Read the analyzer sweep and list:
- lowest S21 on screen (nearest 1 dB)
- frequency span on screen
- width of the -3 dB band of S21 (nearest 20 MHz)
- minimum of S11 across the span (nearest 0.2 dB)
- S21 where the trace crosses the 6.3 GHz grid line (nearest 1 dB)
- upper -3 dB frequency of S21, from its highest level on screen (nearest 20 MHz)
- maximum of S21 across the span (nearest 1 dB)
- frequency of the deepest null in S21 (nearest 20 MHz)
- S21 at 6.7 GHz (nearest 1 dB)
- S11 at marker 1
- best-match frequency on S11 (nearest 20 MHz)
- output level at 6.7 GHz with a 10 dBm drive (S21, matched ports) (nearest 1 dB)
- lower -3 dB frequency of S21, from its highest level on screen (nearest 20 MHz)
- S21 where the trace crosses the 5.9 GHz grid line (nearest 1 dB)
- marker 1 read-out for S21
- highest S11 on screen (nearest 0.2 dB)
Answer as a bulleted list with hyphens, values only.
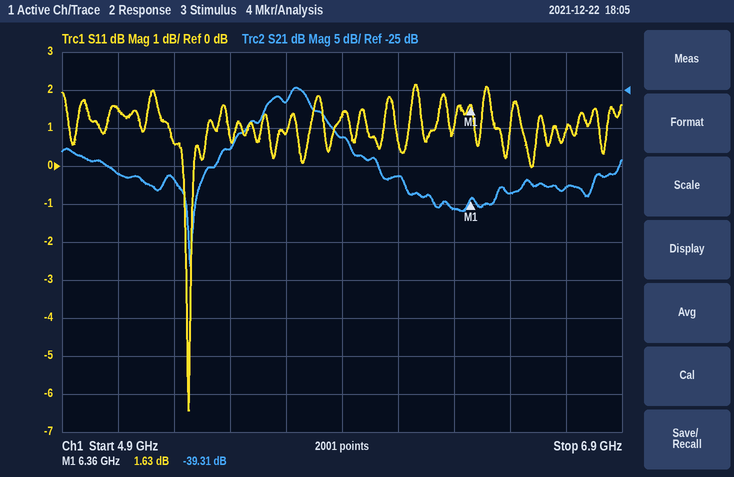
- -48 dB
- 2 GHz
- 180 MHz
- -6.4 dB
- -41 dB
- 5.80 GHz
- -25 dB
- 5.36 GHz
- -38 dB
- 1.63 dB
- 5.36 GHz
- -28 dBm
- 5.62 GHz
- -31 dB
- -39.31 dB
- 2.2 dB
